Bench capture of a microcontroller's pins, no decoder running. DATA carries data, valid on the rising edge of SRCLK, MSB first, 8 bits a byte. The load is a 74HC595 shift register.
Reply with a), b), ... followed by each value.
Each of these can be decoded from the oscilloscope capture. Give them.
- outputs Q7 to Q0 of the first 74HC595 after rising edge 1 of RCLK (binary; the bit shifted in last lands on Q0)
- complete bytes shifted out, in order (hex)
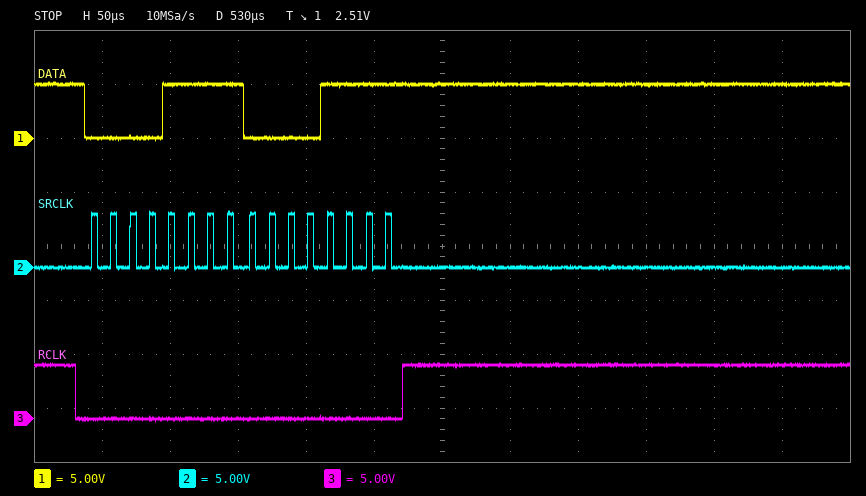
a) 00001111
b) 0F 0F
